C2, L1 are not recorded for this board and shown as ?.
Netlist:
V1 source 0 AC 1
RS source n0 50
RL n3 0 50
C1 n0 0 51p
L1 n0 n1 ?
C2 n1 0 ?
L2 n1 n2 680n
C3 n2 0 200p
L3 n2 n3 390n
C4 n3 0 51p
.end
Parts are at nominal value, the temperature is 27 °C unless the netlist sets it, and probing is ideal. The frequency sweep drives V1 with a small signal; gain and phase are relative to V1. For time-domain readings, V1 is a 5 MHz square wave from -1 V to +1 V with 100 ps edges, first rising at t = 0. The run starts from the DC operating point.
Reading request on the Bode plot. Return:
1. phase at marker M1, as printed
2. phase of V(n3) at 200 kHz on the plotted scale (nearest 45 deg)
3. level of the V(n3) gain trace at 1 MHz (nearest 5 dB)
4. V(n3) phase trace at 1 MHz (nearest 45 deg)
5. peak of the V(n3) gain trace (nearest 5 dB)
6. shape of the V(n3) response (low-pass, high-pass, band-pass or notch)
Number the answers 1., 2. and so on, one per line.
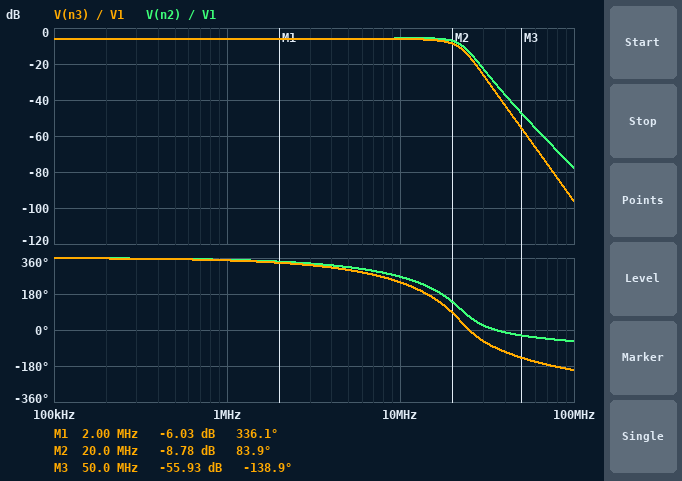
1. 336.1 deg
2. 360 deg
3. -5 dB
4. 360 deg
5. -5 dB
6. low-pass
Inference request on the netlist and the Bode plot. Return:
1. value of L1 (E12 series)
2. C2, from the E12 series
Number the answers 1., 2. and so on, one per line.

1. 820 nH
2. 270 pF
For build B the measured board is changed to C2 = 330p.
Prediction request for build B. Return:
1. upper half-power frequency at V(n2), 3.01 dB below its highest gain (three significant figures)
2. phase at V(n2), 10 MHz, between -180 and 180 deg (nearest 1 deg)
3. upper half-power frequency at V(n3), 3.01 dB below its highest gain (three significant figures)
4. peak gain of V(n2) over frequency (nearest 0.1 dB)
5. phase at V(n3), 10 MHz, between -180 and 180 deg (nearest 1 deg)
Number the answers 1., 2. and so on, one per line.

1. 19.2 MHz
2. -102 deg
3. 17.8 MHz
4. -5.8 dB
5. -130 deg
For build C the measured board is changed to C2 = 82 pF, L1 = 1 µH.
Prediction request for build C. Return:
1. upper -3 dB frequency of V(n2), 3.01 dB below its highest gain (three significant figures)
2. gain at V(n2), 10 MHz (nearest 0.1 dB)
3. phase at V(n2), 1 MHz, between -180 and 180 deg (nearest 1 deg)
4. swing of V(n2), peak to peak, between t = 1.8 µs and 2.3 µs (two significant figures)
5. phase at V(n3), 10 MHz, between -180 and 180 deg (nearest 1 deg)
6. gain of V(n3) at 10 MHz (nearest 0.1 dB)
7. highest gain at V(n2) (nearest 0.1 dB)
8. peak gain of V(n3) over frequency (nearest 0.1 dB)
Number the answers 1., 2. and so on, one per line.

1. 32.3 MHz
2. -7.1 dB
3. -8 deg
4. 1.1 V
5. -104 deg
6. -7.5 dB
7. -2.4 dB
8. -6.0 dB
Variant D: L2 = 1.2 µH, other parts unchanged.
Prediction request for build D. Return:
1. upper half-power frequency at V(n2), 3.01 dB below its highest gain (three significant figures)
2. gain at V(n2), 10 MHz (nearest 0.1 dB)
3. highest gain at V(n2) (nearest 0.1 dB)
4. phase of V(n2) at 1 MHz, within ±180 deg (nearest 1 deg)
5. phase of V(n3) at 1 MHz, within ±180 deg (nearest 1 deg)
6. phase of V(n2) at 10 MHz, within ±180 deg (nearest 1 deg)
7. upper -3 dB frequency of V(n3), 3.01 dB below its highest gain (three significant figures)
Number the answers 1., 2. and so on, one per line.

1. 17.1 MHz
2. -5.9 dB
3. -5.6 dB
4. -11 deg
5. -14 deg
6. -111 deg
7. 16.6 MHz
